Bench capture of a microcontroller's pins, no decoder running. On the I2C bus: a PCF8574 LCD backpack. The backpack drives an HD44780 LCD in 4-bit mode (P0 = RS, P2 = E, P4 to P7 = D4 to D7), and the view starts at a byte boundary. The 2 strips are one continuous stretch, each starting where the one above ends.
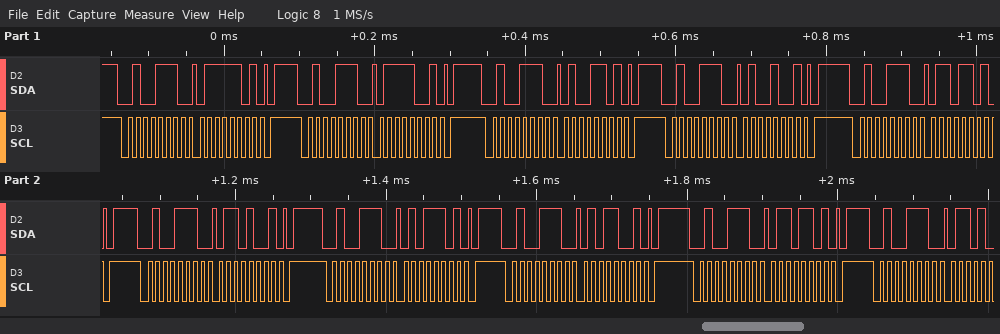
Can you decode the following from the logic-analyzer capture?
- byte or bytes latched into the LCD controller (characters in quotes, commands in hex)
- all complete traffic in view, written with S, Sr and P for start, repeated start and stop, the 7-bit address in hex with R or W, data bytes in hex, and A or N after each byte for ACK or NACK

't' 'e'
S 27W A 7D A P S 27W A 79 A P S 27W A 4D A P S 27W A 49 A P S 27W A 6D A P S 27W A 69 A P S 27W A 5D A P S 27W A 59 A P S 27W A 6D A P S 27W A
